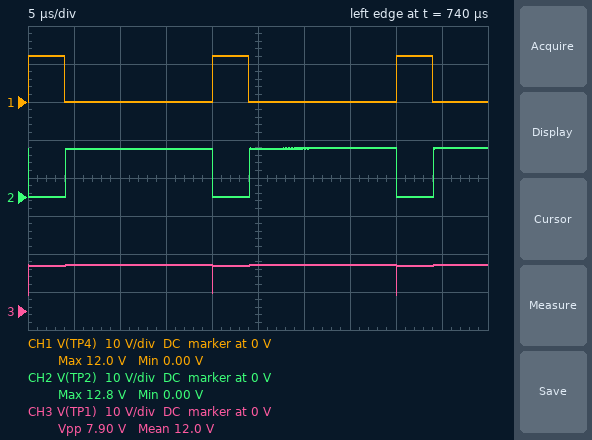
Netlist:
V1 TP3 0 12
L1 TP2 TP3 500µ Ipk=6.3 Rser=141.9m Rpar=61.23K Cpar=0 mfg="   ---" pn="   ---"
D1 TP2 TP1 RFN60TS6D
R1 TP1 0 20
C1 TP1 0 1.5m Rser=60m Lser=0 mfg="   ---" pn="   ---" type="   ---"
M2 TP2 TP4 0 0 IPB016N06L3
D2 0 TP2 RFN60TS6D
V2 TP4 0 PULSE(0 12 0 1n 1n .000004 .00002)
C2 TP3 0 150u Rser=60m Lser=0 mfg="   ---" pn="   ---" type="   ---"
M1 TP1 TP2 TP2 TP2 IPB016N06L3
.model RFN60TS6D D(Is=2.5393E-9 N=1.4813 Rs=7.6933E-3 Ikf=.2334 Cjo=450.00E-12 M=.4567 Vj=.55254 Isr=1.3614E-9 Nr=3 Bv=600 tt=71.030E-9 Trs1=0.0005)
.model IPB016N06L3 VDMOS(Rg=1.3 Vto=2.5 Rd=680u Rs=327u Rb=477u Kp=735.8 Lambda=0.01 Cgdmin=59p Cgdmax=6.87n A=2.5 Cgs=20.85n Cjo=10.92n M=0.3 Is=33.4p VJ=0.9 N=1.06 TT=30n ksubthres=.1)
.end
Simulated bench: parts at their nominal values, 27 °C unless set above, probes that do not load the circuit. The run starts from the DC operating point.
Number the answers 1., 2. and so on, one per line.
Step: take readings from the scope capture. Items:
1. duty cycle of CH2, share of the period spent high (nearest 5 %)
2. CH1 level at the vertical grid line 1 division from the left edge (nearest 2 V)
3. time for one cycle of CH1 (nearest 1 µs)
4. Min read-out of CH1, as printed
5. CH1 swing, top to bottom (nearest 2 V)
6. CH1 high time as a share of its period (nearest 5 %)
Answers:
1. 80 %
2. 0 V
3. 20 µs
4. 0.00 V
5. 12 V
6. 20 %
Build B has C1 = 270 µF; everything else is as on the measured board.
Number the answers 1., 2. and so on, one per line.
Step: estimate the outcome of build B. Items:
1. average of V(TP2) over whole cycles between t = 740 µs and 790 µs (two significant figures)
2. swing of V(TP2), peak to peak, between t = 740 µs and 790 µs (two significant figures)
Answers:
1. 12 V
2. 15 V
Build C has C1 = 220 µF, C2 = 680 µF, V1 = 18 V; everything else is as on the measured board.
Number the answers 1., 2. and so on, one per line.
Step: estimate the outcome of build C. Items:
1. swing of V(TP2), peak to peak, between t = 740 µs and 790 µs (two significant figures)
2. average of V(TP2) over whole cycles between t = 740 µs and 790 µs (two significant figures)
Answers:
1. 23 V
2. 18 V
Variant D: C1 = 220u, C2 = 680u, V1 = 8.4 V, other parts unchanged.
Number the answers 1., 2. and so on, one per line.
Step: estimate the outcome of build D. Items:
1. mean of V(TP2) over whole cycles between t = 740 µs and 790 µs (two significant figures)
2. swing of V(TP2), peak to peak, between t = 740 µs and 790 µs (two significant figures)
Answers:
1. 8.5 V
2. 11 V
